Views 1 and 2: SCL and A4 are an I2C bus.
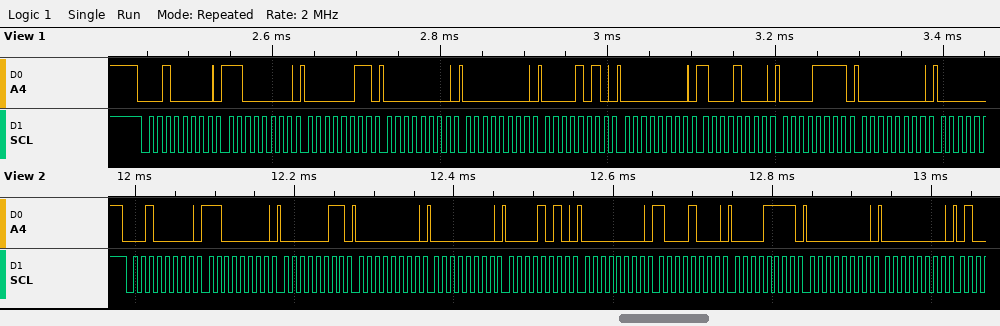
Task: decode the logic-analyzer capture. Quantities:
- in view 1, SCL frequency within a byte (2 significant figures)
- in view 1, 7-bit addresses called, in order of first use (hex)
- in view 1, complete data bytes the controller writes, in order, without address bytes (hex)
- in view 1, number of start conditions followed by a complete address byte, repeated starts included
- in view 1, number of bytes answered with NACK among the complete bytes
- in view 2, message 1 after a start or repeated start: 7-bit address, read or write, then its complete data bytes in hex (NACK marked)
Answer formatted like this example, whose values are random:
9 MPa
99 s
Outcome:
100 kHz
0x10
C0 03 00 00 0A 00 88 0F 00
1
0
0x10 write: C0 03 00 00 0A 00 88 0F 00 00
